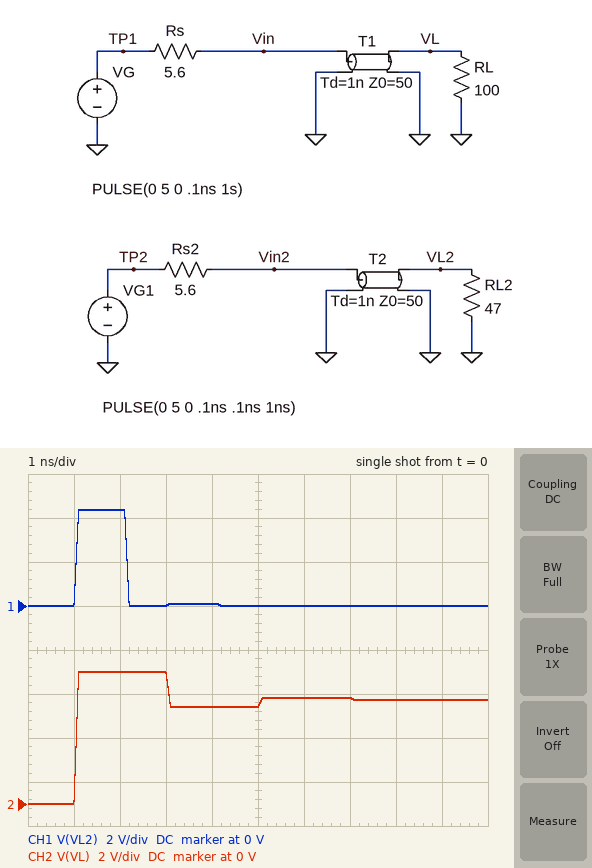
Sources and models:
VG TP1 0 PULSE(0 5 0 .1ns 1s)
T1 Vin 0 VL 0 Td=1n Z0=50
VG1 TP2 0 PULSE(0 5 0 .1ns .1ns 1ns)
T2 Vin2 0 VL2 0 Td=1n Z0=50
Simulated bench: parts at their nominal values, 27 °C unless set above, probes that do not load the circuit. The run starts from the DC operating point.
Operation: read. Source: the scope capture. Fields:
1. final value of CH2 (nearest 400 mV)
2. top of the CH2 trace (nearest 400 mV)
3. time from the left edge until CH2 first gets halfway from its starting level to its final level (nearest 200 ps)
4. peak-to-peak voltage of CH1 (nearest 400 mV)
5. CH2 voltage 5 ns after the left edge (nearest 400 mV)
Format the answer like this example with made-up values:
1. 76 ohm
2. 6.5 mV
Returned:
1. 4.8 V
2. 6.0 V
3. 1.0 ns
4. 4.4 V
5. 4.4 V
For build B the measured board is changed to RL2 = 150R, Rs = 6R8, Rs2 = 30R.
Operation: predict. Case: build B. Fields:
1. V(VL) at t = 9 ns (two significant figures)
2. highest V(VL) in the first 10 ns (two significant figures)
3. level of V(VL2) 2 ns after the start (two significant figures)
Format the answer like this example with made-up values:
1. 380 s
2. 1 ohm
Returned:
1. 4.7 V
2. 5.9 V
3. 4.7 V
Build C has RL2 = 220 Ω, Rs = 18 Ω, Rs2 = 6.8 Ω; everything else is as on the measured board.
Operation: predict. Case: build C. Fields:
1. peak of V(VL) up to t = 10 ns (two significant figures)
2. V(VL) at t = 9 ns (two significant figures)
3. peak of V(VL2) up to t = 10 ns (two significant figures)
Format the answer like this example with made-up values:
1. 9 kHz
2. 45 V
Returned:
1. 4.9 V
2. 4.2 V
3. 7.2 V
